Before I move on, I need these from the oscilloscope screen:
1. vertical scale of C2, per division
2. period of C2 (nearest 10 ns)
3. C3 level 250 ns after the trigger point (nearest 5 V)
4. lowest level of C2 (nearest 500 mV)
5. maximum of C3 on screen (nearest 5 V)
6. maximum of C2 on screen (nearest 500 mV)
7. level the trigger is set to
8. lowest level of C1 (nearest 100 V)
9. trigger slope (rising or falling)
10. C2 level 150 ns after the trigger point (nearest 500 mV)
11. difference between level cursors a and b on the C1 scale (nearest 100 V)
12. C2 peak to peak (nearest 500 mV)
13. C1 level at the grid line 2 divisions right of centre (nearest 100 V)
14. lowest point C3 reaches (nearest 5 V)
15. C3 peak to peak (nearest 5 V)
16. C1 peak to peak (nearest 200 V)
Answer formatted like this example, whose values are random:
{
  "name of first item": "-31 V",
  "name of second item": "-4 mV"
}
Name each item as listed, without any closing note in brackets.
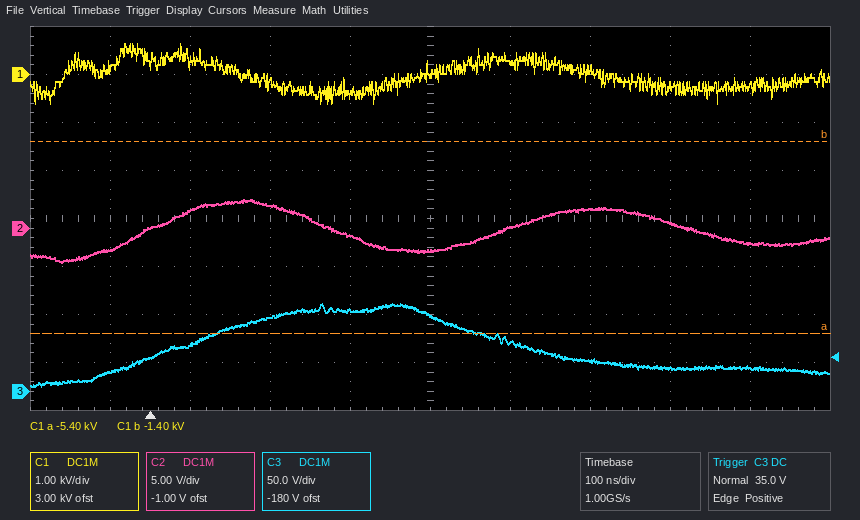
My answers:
{
  "vertical scale of C2, per division": "5 V",
  "period of C2": "450 ns",
  "C3 level 250 ns after the trigger point": "85 V",
  "lowest level of C2": "-3.5 V",
  "maximum of C3 on screen": "90 V",
  "maximum of C2 on screen": "3.0 V",
  "level the trigger is set to": "35.0 V",
  "lowest level of C1": "-600 V",
  "trigger slope": "rising",
  "C2 level 150 ns after the trigger point": "2.5 V",
  "difference between level cursors a and b on the C1 scale": "4.0 kV",
  "C2 peak to peak": "6.5 V",
  "C1 level at the grid line 2 divisions right of centre": "100 V",
  "lowest point C3 reaches": "5 V",
  "C3 peak to peak": "85 V",
  "C1 peak to peak": "1.2 kV"
}
